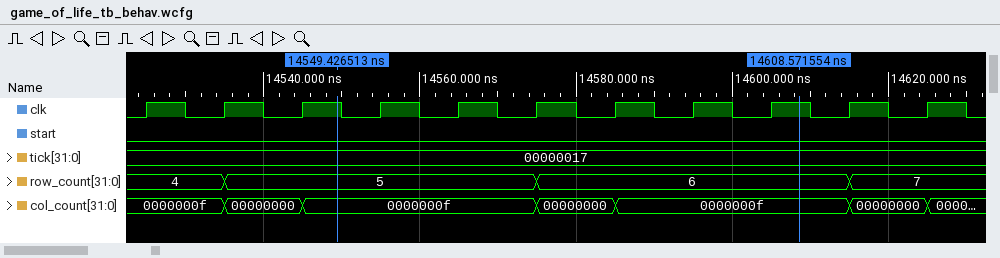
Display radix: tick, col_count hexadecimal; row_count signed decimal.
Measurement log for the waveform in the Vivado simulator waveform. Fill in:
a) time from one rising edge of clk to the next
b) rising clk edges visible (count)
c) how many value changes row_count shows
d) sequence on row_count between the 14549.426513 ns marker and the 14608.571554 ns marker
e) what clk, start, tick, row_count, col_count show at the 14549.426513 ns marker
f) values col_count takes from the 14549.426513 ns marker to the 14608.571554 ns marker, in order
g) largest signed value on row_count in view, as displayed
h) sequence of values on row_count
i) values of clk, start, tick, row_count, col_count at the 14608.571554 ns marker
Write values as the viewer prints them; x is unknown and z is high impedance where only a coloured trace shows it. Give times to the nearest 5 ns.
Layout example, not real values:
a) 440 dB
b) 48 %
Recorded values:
a) 10 ns
b) 11
c) 3
d) 5, 6
e) clk=1, start=0, tick=00000017, row_count=5, col_count=0000000f
f) 0000000f, 00000000, 0000000f
g) 7
h) 4, 5, 6, 7
i) clk=1, start=0, tick=00000017, row_count=6, col_count=0000000f
